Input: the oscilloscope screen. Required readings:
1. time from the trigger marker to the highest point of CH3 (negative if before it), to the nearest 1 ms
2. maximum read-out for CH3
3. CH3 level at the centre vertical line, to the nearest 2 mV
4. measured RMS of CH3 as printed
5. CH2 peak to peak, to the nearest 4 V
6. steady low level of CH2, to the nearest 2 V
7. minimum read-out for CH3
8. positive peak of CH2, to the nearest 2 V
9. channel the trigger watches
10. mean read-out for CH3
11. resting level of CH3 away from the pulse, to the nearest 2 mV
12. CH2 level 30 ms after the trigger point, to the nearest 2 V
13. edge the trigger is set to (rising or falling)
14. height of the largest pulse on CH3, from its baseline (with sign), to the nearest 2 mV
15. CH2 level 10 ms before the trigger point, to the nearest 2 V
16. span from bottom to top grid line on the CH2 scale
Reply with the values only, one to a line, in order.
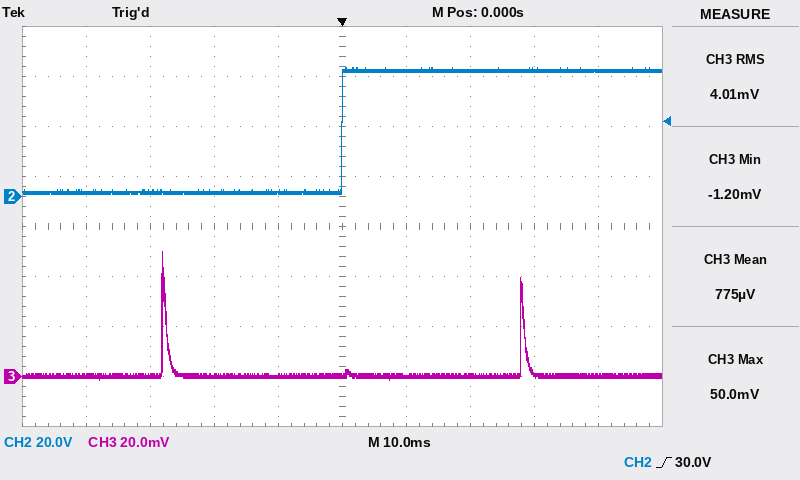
-28 ms
50.0 mV
0 mV
4.01 mV
52 V
2 V
-1.20 mV
52 V
CH2
775 µV
0 mV
50 V
rising
+50 mV
2 V
160 V
